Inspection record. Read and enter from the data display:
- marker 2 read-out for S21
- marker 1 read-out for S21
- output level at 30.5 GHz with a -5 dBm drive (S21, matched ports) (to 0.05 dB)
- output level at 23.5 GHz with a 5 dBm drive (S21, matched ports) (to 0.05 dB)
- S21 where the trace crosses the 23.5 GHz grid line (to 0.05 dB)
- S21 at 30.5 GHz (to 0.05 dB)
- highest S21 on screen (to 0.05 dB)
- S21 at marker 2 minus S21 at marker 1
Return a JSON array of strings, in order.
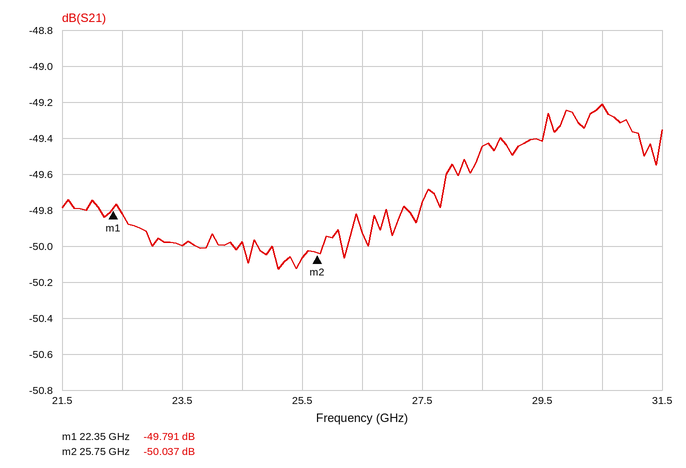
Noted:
["-50.037 dB", "-49.791 dB", "-54.20 dBm", "-45.00 dBm", "-50.00 dB", "-49.20 dB", "-49.20 dB", "-0.246 dB"]
